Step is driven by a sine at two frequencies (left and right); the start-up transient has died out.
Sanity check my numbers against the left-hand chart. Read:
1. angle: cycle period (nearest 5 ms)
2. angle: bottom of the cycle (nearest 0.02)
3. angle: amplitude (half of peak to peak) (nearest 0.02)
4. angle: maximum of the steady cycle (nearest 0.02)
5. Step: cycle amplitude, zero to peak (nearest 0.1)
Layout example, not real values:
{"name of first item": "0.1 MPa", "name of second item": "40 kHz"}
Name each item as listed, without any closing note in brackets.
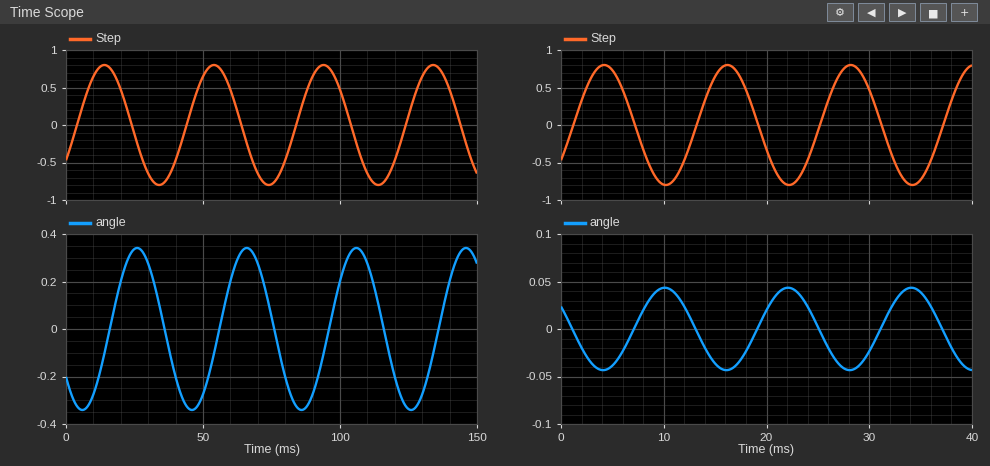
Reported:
{"angle: cycle period": "40 ms", "angle: bottom of the cycle": "-0.34", "angle: amplitude (half of peak to peak)": "0.34", "angle: maximum of the steady cycle": "0.34", "Step: cycle amplitude, zero to peak": "0.8"}
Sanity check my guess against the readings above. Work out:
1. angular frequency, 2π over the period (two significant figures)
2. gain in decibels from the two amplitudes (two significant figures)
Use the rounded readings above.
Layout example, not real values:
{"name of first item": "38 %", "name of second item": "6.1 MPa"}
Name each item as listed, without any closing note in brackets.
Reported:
{"angular frequency, 2π over the period": "0.16 rad/ms", "gain in decibels from the two amplitudes": "-7.4 dB"}
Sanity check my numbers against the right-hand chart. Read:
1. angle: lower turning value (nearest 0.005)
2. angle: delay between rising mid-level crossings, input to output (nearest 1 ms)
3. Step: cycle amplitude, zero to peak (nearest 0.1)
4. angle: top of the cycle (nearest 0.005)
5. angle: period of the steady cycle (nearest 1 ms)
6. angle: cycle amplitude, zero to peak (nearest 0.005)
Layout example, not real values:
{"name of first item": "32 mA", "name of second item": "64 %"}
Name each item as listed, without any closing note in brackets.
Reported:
{"angle: lower turning value": "-0.045", "angle: delay between rising mid-level crossings, input to output": "6 ms", "Step: cycle amplitude, zero to peak": "0.8", "angle: top of the cycle": "0.045", "angle: period of the steady cycle": "12 ms", "angle: cycle amplitude, zero to peak": "0.045"}
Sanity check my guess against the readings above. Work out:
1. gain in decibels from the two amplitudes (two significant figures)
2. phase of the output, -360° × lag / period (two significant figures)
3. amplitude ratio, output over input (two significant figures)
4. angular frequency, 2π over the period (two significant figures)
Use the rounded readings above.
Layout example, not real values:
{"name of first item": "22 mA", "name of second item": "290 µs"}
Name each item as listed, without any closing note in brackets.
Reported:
{"gain in decibels from the two amplitudes": "-25 dB", "phase of the output, -360° × lag / period": "-180°", "amplitude ratio, output over input": "0.056", "angular frequency, 2π over the period": "0.52 rad/ms"}
